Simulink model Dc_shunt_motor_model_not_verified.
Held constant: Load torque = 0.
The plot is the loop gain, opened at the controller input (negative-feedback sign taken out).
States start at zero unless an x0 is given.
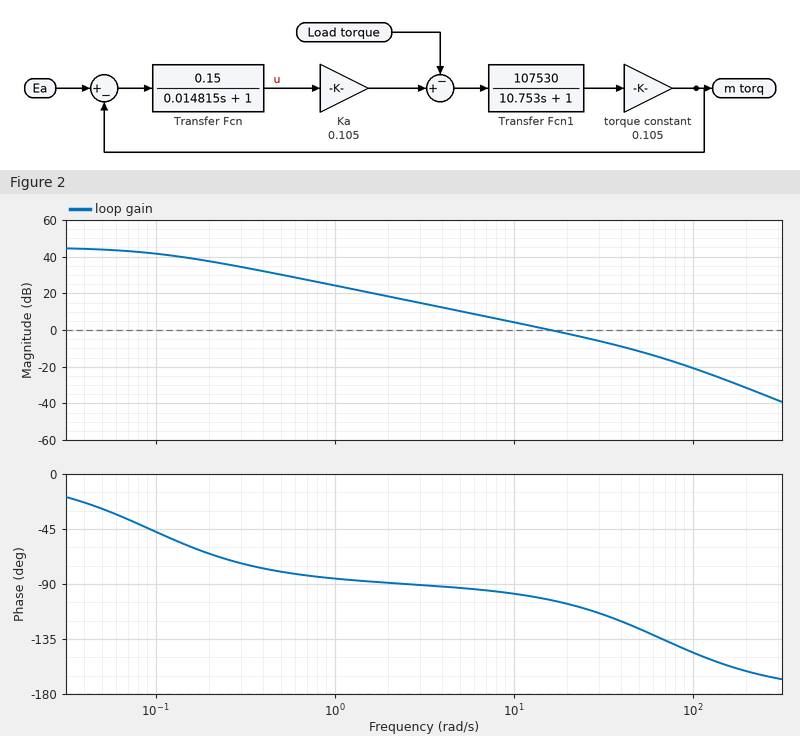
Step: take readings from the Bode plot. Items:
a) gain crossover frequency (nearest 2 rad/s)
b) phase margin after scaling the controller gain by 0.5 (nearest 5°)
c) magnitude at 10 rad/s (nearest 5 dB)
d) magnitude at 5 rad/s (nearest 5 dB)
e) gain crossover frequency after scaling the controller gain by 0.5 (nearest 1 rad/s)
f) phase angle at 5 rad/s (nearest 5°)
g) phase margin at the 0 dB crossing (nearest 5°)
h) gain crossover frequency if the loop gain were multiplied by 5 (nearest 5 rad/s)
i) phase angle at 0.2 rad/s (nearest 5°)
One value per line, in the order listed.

16 rad/s
85°
5 dB
10 dB
8 rad/s
-95°
75°
60 rad/s
-65°
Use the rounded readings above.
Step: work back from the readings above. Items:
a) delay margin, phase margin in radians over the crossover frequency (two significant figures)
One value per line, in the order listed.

0.082 s
